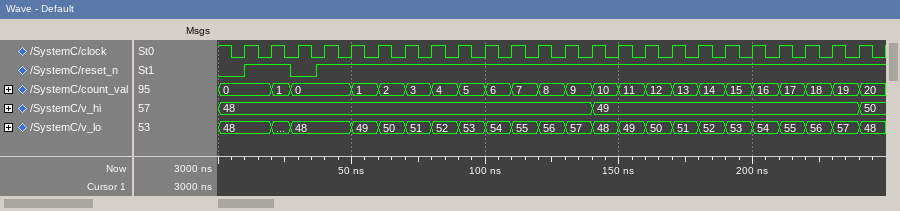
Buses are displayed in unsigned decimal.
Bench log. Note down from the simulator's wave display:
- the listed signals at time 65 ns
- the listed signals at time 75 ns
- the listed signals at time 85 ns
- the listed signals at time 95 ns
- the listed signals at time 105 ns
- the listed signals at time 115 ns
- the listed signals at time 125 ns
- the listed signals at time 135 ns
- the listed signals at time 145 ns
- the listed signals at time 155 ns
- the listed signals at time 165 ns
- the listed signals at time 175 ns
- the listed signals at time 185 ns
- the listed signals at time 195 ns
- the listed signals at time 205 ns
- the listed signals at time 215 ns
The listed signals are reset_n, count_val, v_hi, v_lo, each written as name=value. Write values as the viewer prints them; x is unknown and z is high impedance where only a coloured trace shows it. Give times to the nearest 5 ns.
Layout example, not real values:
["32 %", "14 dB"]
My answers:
["reset_n=1, count_val=2, v_hi=48, v_lo=50", "reset_n=1, count_val=3, v_hi=48, v_lo=51", "reset_n=1, count_val=4, v_hi=48, v_lo=52", "reset_n=1, count_val=5, v_hi=48, v_lo=53", "reset_n=1, count_val=6, v_hi=48, v_lo=54", "reset_n=1, count_val=7, v_hi=48, v_lo=55", "reset_n=1, count_val=8, v_hi=48, v_lo=56", "reset_n=1, count_val=9, v_hi=48, v_lo=57", "reset_n=1, count_val=10, v_hi=49, v_lo=48", "reset_n=1, count_val=11, v_hi=49, v_lo=49", "reset_n=1, count_val=12, v_hi=49, v_lo=50", "reset_n=1, count_val=13, v_hi=49, v_lo=51", "reset_n=1, count_val=14, v_hi=49, v_lo=52", "reset_n=1, count_val=15, v_hi=49, v_lo=53", "reset_n=1, count_val=16, v_hi=49, v_lo=54", "reset_n=1, count_val=17, v_hi=49, v_lo=55"]
